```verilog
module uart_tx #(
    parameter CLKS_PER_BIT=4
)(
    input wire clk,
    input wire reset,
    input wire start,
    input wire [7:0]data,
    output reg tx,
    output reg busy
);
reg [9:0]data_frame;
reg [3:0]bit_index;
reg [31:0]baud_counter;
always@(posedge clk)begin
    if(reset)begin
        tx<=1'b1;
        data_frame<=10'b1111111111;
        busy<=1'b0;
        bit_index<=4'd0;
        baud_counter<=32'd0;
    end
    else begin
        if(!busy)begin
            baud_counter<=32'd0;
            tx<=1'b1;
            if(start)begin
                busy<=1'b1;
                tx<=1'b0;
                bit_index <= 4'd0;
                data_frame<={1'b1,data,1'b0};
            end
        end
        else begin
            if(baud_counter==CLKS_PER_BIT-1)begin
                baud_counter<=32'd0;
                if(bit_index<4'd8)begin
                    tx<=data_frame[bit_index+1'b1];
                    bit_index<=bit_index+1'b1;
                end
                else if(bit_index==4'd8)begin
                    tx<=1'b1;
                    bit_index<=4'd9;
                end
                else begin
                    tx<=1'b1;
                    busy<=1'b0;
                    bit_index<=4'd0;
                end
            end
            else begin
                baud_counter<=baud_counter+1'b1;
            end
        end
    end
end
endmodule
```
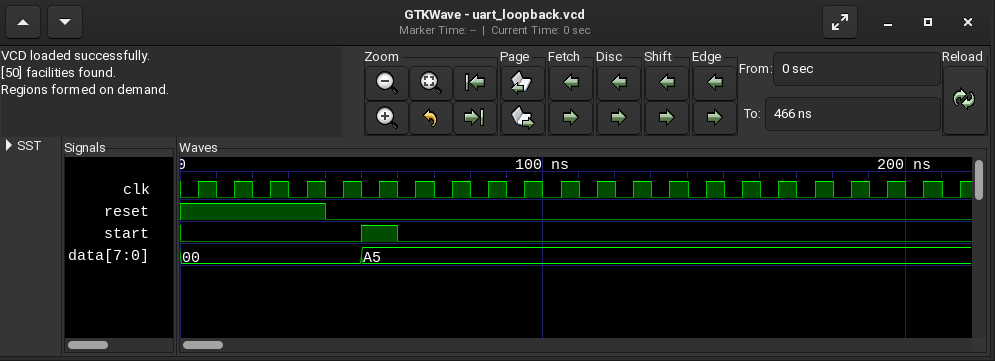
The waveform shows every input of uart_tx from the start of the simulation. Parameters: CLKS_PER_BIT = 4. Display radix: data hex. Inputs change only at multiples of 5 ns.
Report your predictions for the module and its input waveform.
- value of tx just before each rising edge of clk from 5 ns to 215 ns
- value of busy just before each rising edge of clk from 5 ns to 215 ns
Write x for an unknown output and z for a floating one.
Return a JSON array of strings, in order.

["x 1 1 1 1 1 0 0 0 0 1 1 1 1 0 0 0 0 1 1 1 1", "x 0 0 0 0 0 1 1 1 1 1 1 1 1 1 1 1 1 1 1 1 1"]
